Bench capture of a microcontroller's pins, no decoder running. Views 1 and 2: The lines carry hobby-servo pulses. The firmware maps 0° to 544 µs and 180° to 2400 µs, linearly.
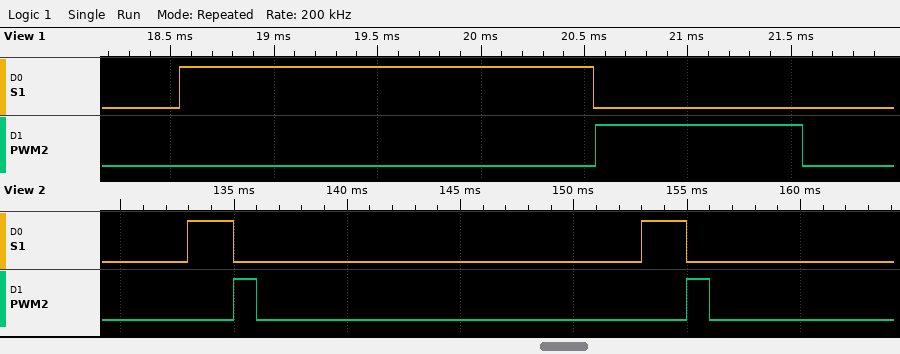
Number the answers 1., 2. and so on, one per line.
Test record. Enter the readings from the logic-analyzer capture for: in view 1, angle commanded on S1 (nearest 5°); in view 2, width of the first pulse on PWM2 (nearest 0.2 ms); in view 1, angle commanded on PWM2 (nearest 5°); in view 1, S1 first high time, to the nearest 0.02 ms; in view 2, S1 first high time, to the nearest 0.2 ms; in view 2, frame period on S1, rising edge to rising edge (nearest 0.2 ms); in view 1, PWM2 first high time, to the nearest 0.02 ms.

1. 140°
2. 1.0 ms
3. 45°
4. 2.00 ms
5. 2.0 ms
6. 20.0 ms
7. 1.00 ms
